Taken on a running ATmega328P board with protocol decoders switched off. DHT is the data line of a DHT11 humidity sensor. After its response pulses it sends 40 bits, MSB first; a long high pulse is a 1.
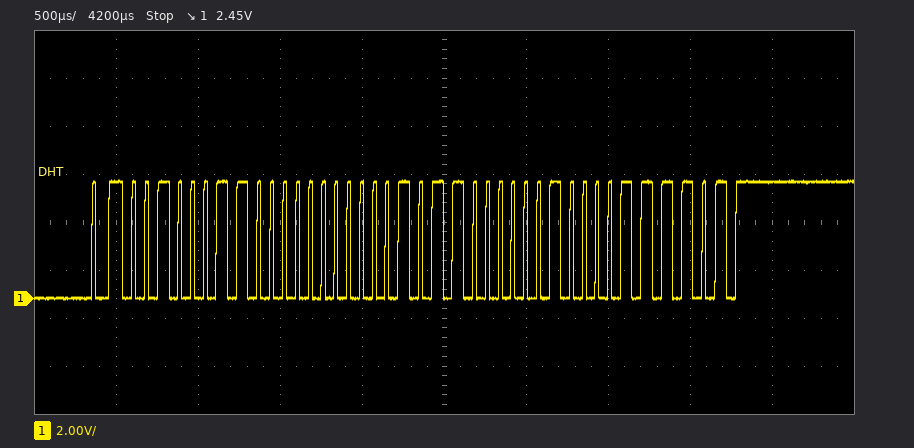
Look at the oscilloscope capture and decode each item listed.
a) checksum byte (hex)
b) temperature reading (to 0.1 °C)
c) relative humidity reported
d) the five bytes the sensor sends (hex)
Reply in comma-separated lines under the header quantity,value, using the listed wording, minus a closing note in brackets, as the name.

quantity,value
checksum byte,0x3D
temperature reading,22.4 °C
relative humidity reported,35 %
the five bytes the sensor sends,23 00 16 04 3D
